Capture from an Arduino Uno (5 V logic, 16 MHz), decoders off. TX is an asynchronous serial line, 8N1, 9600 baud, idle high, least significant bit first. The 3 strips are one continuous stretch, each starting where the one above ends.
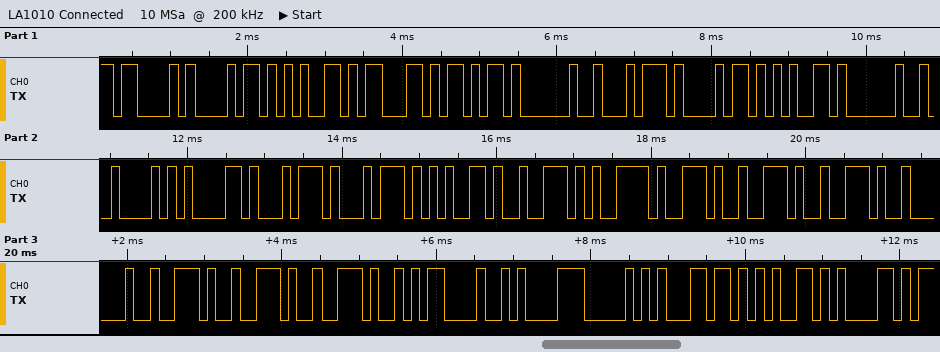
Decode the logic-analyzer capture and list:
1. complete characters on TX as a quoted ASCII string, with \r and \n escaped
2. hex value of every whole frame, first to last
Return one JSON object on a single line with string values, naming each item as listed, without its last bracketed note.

{"complete characters on TX as a quoted ASCII string, with \\r and \\n escaped": "\"Check the Battery... ...\\r\\nPlea\"", "hex value of every whole frame, first to last": "43 68 65 63 6B 20 74 68 65 20 42 61 74 74 65 72 79 2E 2E 2E 20 2E 2E 2E 0D 0A 50 6C 65 61"}
